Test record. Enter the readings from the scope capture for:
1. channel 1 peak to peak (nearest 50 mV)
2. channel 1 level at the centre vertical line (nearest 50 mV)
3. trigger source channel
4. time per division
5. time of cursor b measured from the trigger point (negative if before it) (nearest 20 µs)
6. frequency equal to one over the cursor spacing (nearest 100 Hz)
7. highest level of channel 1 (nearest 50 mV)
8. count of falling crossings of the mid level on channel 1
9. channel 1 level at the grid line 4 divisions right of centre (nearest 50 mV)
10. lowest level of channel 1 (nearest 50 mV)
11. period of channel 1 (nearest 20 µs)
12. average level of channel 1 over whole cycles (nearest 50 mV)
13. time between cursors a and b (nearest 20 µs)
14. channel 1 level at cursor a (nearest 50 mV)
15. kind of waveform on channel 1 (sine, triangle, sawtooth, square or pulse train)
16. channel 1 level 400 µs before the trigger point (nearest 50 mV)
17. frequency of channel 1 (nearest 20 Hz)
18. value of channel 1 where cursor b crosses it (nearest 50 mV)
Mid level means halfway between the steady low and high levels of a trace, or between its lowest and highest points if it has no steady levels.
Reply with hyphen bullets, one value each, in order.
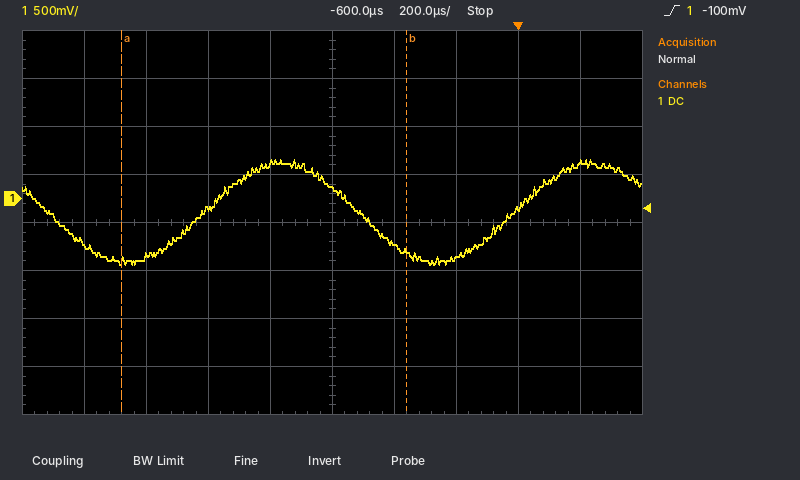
- 1.10 V
- 100 mV
- channel 1
- 200 µs
- -360 µs
- 1.1 kHz
- 400 mV
- 2
- 350 mV
- -700 mV
- 1.00 ms
- -150 mV
- 920 µs
- -650 mV
- sine
- -450 mV
- 1.00 kHz
- -550 mV
